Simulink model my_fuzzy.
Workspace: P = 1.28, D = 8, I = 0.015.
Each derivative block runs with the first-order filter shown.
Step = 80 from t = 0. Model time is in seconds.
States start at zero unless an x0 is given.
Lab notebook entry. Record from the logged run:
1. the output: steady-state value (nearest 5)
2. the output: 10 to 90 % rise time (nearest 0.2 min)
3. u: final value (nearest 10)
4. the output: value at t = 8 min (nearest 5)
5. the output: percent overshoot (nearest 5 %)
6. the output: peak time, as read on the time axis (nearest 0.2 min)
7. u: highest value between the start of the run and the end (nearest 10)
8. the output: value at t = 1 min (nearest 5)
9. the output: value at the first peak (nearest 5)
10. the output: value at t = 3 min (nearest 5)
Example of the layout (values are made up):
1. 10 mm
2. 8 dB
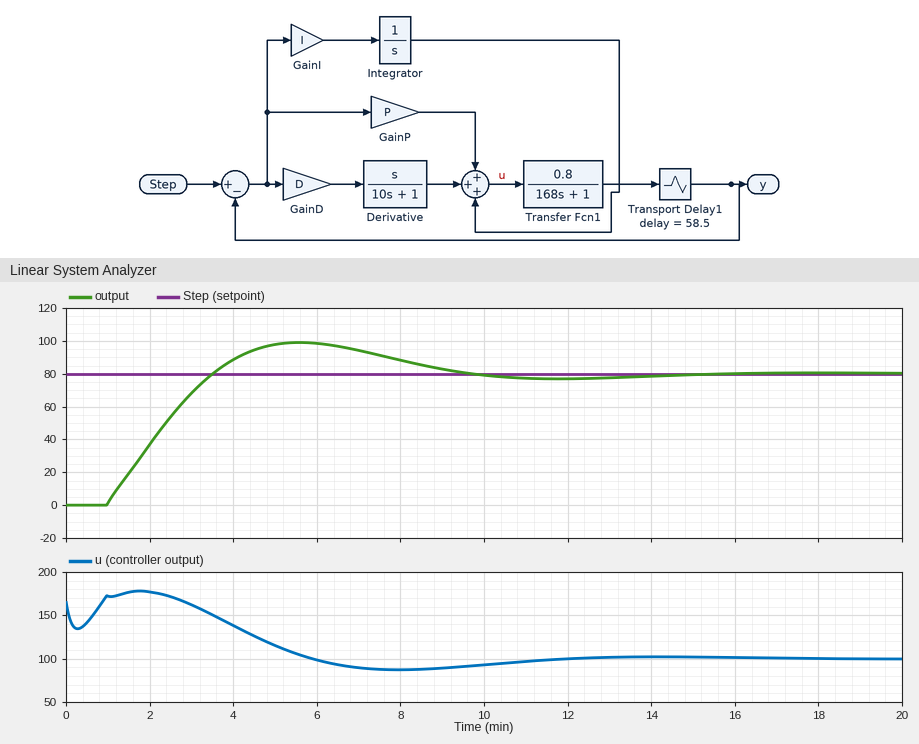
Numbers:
1. 80
2. 2.0 min
3. 100
4. 90
5. 25 %
6. 5.6 min
7. 180
8. 0
9. 100
10. 70
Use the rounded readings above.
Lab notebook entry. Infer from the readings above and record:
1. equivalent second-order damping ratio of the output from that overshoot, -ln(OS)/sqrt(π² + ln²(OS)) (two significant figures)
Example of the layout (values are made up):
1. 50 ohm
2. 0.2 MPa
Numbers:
1. 0.40
